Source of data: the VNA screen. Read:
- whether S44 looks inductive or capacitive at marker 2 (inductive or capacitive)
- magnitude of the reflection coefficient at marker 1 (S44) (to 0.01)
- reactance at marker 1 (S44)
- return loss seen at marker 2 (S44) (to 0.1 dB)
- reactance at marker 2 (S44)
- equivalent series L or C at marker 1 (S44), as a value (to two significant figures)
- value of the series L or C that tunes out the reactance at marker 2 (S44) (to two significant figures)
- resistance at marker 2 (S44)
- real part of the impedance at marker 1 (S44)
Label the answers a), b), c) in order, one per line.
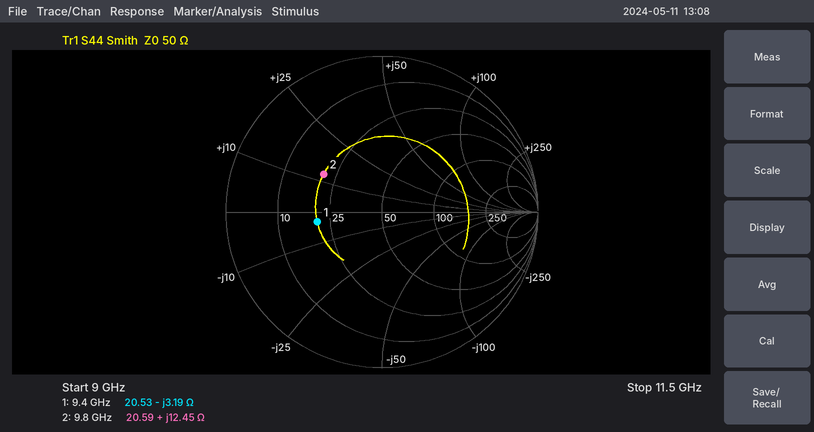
a) inductive
b) 0.42
c) -3.19 Ω
d) 7.0 dB
e) +12.45 Ω
f) 5.3 pF
g) 1.3 pF
h) 20.59 Ω
i) 20.53 Ω
